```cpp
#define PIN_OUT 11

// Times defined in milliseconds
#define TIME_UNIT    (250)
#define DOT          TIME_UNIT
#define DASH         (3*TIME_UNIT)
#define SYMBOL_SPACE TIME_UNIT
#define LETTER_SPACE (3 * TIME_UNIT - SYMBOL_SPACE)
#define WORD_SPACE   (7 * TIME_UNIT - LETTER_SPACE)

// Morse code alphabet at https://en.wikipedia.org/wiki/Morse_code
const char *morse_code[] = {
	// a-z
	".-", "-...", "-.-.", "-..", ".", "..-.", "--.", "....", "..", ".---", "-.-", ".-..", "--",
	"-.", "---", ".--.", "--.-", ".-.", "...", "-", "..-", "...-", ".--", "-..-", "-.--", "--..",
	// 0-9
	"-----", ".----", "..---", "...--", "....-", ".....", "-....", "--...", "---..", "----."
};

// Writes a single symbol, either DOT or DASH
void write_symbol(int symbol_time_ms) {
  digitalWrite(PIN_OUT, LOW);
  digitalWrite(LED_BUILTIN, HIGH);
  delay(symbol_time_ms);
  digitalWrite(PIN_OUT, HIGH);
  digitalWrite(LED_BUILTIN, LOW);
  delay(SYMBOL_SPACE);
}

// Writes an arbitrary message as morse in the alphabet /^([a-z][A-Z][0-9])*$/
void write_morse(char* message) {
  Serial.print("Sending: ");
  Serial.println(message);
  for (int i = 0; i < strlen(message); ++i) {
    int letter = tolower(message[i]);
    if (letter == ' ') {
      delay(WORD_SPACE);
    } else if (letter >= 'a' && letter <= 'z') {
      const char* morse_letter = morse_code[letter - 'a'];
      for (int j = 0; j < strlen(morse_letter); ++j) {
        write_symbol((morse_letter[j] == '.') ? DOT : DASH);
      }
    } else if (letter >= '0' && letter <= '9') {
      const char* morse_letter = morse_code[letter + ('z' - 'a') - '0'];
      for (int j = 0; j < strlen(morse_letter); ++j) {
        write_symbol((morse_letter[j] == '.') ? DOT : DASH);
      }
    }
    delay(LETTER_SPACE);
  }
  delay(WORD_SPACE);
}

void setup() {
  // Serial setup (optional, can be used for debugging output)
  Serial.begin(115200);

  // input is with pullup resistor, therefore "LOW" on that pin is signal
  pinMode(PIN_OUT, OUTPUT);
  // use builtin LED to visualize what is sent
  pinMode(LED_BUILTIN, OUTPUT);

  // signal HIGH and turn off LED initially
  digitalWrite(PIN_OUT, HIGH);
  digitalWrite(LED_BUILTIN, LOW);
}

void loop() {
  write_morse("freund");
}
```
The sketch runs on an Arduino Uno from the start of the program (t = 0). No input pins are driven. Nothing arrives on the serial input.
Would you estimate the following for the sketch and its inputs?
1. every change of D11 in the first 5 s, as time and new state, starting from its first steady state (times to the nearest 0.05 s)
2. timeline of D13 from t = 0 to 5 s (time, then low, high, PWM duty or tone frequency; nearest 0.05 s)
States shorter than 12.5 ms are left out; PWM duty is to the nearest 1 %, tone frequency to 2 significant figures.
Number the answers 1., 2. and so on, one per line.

1. 0 s low; 0.25 s high; 0.5 s low; 0.75 s high; 1 s low; 1.75 s high; 2 s low; 2.25 s high; 3 s low; 3.25 s high; 3.5 s low; 4.25 s high; 4.5 s low; 4.75 s high
2. 0 s high; 0.25 s low; 0.5 s high; 0.75 s low; 1 s high; 1.75 s low; 2 s high; 2.25 s low; 3 s high; 3.25 s low; 3.5 s high; 4.25 s low; 4.5 s high; 4.75 s low
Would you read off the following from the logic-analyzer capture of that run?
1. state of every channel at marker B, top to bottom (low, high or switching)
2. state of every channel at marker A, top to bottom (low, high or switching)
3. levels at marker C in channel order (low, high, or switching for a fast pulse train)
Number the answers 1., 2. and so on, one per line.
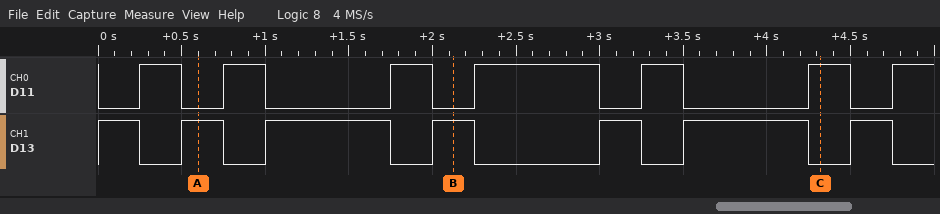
1. D11 low, D13 high
2. D11 low, D13 high
3. D11 high, D13 low
